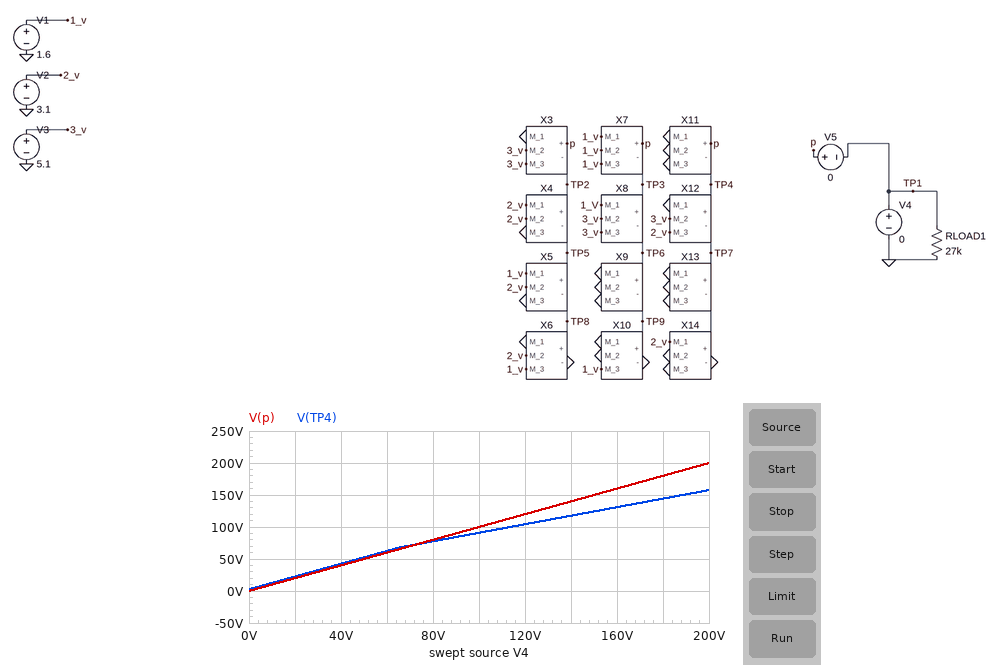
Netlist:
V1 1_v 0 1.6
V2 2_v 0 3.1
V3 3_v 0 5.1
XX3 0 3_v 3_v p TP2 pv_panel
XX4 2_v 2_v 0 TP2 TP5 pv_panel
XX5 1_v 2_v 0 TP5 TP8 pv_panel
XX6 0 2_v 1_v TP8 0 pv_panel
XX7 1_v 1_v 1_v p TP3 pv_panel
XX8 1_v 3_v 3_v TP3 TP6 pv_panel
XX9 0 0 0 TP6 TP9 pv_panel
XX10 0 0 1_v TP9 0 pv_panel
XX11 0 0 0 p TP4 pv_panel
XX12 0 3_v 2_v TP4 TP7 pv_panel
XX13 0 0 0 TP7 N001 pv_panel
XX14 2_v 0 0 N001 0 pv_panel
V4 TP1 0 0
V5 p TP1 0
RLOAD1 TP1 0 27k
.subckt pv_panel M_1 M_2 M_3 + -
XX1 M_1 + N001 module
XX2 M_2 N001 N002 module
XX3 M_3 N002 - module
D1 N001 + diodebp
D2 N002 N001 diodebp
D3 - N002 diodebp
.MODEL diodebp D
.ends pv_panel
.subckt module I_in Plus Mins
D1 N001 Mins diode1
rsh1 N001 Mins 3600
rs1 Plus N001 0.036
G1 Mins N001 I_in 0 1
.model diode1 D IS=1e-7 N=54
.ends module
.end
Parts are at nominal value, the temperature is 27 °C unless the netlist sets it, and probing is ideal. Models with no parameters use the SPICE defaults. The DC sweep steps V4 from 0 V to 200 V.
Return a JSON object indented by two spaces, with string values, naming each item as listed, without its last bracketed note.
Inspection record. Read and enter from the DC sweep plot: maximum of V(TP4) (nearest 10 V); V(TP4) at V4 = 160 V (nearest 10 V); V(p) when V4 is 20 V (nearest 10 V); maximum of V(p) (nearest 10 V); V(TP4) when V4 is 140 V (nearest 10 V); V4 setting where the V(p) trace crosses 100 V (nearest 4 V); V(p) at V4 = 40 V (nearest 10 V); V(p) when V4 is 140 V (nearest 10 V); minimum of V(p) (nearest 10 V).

{
  "maximum of V(TP4)": "160 V",
  "V(TP4) at V4 = 160 V": "130 V",
  "V(p) when V4 is 20 V": "20 V",
  "maximum of V(p)": "200 V",
  "V(TP4) when V4 is 140 V": "120 V",
  "V4 setting where the V(p) trace crosses 100 V": "100 V",
  "V(p) at V4 = 40 V": "40 V",
  "V(p) when V4 is 140 V": "140 V",
  "minimum of V(p)": "0 V"
}
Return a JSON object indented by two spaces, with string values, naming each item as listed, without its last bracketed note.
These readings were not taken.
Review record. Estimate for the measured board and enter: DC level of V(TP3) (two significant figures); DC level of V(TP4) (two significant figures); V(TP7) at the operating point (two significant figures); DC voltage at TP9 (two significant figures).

{
  "DC level of V(TP3)": "2.6 V",
  "DC level of V(TP4)": "2.6 V",
  "V(TP7) at the operating point": "-5.2 V",
  "DC voltage at TP9": "-2.6 V"
}
